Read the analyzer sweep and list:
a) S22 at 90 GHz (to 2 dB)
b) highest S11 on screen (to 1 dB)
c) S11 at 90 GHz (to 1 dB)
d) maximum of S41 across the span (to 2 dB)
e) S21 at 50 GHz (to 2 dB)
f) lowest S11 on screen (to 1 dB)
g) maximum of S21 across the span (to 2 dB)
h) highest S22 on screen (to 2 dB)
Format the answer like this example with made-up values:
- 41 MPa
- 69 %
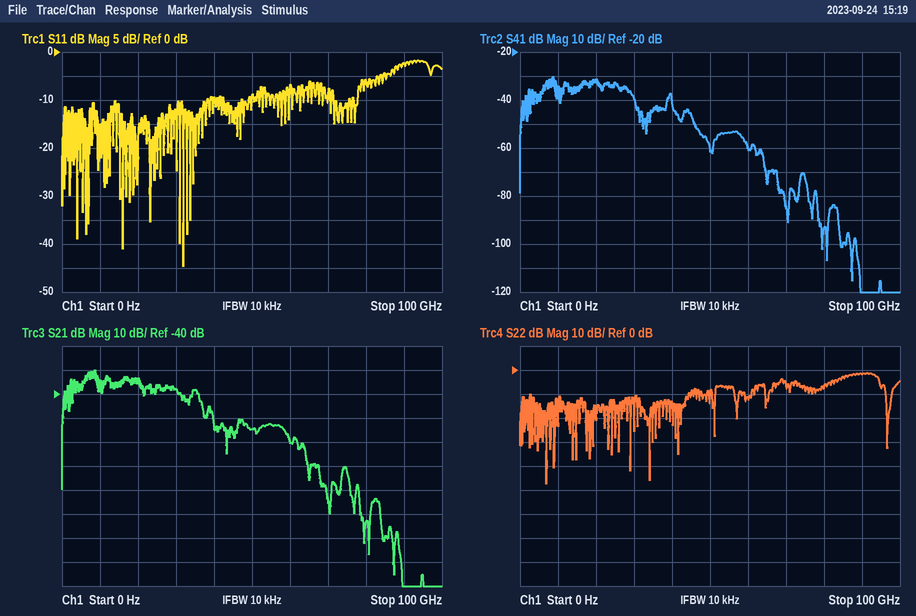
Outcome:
- -2 dB
- -2 dB
- -2 dB
- -30 dB
- -54 dB
- -45 dB
- -30 dB
- -2 dB
